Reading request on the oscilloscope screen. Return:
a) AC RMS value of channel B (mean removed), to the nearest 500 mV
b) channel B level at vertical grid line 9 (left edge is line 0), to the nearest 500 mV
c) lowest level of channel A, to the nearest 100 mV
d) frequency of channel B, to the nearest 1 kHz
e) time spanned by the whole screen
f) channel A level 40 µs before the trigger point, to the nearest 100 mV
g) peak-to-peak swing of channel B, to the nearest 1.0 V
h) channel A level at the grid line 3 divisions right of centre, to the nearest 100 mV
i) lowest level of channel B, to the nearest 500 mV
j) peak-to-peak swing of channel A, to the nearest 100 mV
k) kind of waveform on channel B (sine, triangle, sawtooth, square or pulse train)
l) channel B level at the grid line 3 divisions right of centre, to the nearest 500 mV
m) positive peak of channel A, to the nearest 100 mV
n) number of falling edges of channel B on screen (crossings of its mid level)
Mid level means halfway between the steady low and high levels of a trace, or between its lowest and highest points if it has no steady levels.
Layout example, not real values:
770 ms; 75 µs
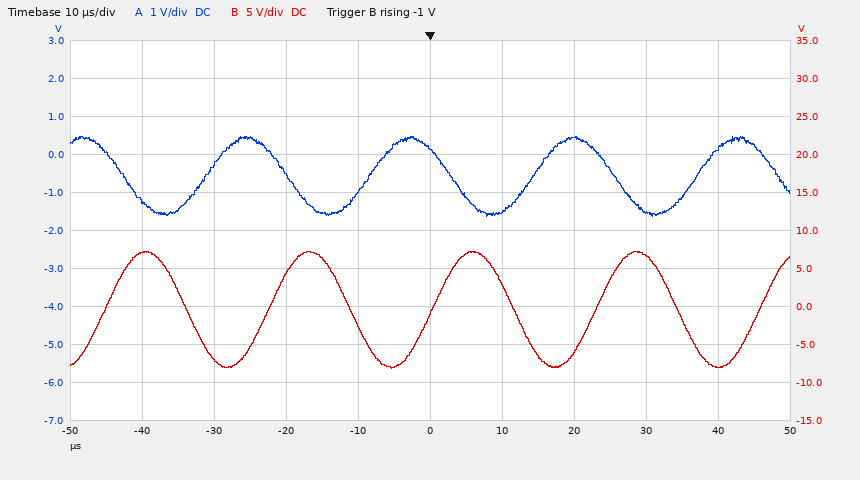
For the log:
5.5 V; -8.0 V; -1.6 V; 44 kHz; 100 µs; -1.2 V; 15.0 V; -1.5 V; -8.0 V; 2.1 V; sine; 6.5 V; 500 mV; 4
